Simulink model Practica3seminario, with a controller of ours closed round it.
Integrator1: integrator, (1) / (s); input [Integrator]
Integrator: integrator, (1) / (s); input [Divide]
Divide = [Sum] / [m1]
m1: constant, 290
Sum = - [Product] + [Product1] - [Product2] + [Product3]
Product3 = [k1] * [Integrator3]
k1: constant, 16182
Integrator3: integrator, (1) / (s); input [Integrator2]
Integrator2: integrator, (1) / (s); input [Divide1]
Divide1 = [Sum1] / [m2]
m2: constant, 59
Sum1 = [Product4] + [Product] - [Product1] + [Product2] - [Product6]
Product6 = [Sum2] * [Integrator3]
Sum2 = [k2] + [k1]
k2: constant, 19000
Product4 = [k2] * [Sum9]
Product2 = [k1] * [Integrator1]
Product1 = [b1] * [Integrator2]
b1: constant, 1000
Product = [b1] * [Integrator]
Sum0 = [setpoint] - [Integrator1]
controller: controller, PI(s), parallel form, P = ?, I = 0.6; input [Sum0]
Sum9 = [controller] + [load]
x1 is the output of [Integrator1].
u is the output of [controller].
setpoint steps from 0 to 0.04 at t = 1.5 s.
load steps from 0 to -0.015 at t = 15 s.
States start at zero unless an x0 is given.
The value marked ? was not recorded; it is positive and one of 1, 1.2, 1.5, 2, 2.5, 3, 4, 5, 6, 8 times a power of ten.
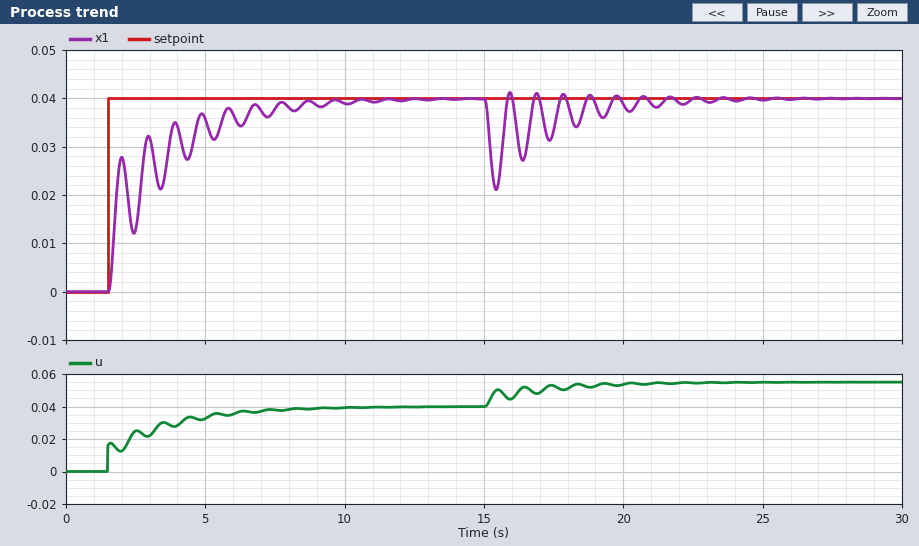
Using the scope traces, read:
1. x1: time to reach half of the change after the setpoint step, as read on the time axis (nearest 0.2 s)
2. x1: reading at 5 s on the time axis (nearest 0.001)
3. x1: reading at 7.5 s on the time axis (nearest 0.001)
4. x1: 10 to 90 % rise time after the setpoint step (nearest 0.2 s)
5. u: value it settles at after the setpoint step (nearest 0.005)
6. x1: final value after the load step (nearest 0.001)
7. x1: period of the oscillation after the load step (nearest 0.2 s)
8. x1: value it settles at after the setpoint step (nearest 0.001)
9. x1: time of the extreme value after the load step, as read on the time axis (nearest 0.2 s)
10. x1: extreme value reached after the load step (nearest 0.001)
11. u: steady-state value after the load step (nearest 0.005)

1.8 s
0.036
0.038
3.2 s
0.040
0.040
1.0 s
0.040
15.4 s
0.021
0.055
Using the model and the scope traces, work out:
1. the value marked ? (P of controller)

0.4
